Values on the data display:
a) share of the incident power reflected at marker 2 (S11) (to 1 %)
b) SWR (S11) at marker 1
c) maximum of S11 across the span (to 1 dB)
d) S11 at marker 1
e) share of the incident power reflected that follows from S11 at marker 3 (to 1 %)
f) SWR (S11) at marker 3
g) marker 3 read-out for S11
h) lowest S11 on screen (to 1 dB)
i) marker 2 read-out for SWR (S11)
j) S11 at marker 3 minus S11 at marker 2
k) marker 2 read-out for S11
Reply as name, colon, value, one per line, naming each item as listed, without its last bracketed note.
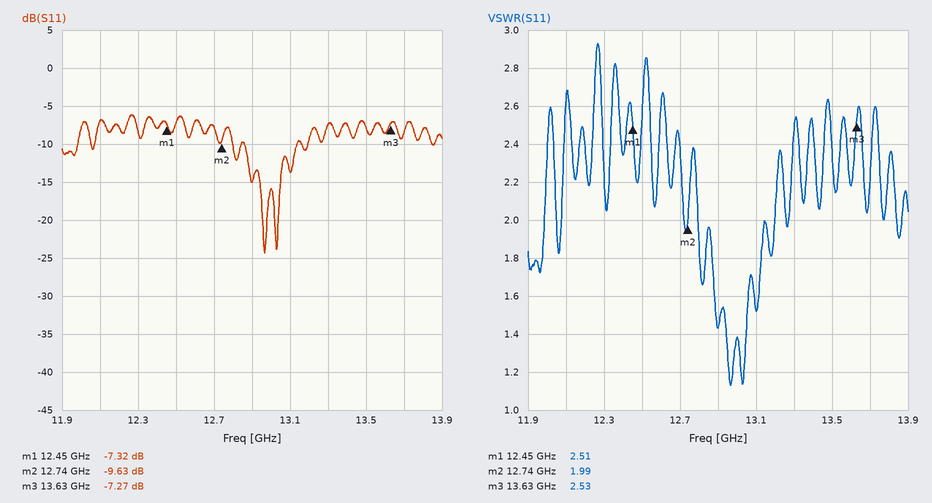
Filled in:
share of the incident power reflected at marker 2 (S11): 11 %
SWR (S11) at marker 1: 2.51
maximum of S11 across the span: -6 dB
S11 at marker 1: -7.32 dB
share of the incident power reflected that follows from S11 at marker 3: 19 %
SWR (S11) at marker 3: 2.53
marker 3 read-out for S11: -7.27 dB
lowest S11 on screen: -24 dB
marker 2 read-out for SWR: 1.99
S11 at marker 3 minus S11 at marker 2: 2.36 dB
marker 2 read-out for S11: -9.63 dB
